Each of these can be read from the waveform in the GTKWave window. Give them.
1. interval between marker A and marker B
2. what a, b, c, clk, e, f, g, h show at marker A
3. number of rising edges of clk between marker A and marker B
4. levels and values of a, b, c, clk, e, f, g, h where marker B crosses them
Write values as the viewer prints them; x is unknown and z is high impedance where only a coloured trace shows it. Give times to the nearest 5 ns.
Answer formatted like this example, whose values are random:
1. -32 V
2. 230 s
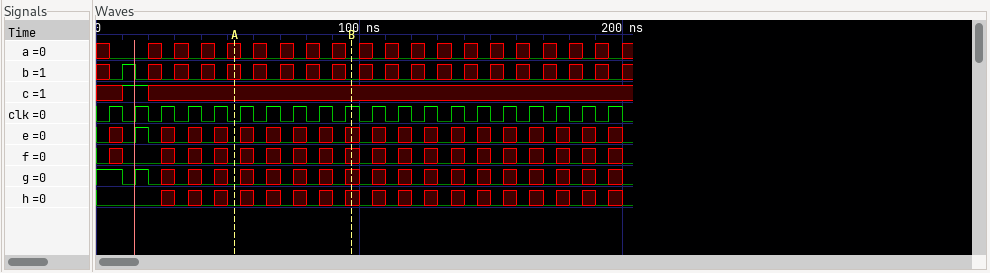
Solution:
1. 45 ns
2. a=x, b=x, c=x, clk=0, e=0, f=0, g=0, h=0
3. 5
4. a=0, b=0, c=x, clk=1, e=x, f=x, g=x, h=x
